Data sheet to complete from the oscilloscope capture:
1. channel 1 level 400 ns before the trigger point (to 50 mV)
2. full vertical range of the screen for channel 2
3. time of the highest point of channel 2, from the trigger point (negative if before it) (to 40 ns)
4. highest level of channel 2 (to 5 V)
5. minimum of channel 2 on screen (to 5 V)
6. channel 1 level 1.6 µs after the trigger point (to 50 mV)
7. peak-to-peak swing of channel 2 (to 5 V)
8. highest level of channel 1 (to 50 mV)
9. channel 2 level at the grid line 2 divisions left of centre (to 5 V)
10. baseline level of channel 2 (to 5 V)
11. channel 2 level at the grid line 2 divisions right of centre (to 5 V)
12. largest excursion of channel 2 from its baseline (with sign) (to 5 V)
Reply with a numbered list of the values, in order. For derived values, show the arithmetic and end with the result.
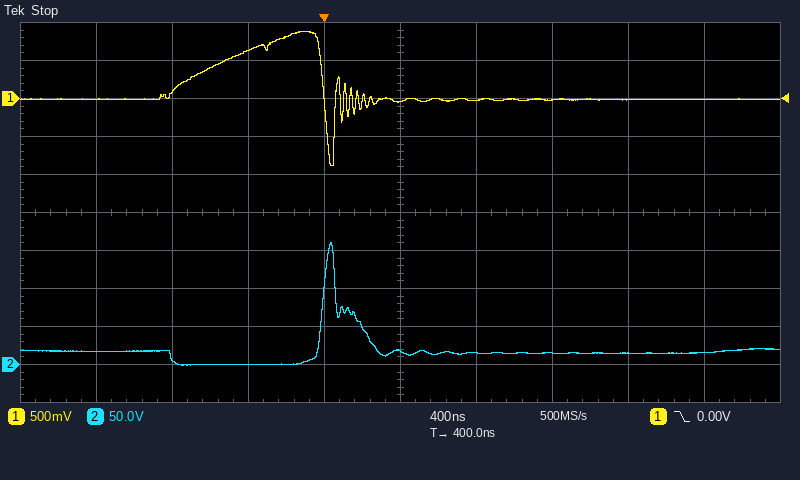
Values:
1. 650 mV
2. 500 V
3. +40 ns
4. 160 V
5. 0 V
6. 0 mV
7. 160 V − (0 V) = 160 V
8. 900 mV
9. 0 V
10. 15 V
11. 15 V
12. 160 V − (15 V) = +145 V
